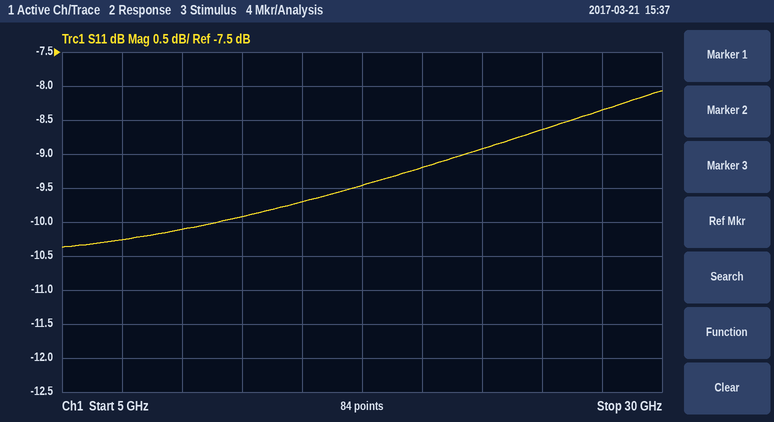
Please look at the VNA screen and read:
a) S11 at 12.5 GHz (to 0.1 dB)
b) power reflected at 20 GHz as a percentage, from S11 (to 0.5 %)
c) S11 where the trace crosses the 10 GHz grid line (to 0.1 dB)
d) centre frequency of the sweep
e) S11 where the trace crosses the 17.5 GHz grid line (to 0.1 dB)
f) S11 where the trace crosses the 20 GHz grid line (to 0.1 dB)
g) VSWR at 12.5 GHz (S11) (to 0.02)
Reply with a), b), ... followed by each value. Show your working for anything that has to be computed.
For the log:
a) -9.9 dB
b) 10^(-9.2/10) ≈ 12.0 %
c) -10.1 dB
d) 17.5 GHz
e) -9.5 dB
f) -9.2 dB
g) |Γ| = 10^(-9.9/20) = 0.3199; VSWR = (1 + 0.3199)/(1 − 0.3199) ≈ 1.94
